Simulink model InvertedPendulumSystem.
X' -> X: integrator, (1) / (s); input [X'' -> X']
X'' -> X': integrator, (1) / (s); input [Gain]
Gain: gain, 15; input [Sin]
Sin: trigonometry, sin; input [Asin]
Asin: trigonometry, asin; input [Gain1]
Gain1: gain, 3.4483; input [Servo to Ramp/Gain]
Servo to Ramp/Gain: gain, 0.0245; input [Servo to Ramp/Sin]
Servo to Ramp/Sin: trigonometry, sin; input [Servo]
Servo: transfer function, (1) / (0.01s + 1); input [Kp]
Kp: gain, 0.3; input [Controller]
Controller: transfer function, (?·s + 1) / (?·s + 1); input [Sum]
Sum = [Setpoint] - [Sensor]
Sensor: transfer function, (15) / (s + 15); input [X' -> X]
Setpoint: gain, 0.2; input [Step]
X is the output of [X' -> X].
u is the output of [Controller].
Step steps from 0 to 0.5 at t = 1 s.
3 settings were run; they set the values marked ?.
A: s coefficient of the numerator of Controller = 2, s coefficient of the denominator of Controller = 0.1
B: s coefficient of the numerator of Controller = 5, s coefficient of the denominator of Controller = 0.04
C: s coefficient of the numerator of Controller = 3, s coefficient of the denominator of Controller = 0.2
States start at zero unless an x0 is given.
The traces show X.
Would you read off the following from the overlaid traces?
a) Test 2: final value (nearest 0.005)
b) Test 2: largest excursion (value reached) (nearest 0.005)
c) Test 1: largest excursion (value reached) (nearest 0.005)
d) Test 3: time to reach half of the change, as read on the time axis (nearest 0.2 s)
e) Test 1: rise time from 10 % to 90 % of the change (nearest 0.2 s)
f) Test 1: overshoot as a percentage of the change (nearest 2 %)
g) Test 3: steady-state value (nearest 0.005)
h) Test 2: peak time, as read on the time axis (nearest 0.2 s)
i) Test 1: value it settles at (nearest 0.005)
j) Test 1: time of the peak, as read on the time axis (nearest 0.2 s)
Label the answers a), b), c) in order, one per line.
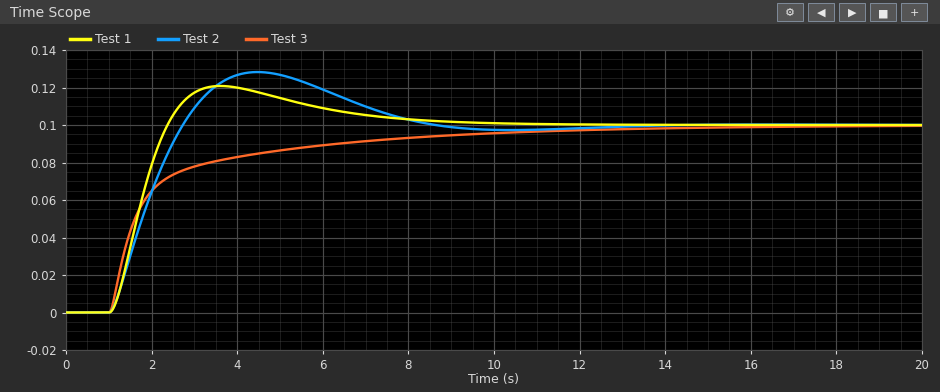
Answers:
a) 0.100
b) 0.130
c) 0.120
d) 1.6 s
e) 1.0 s
f) 20 %
g) 0.100
h) 4.4 s
i) 0.100
j) 3.6 s
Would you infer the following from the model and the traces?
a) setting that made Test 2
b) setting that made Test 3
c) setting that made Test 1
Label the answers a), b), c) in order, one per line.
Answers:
a) A
b) B
c) C
